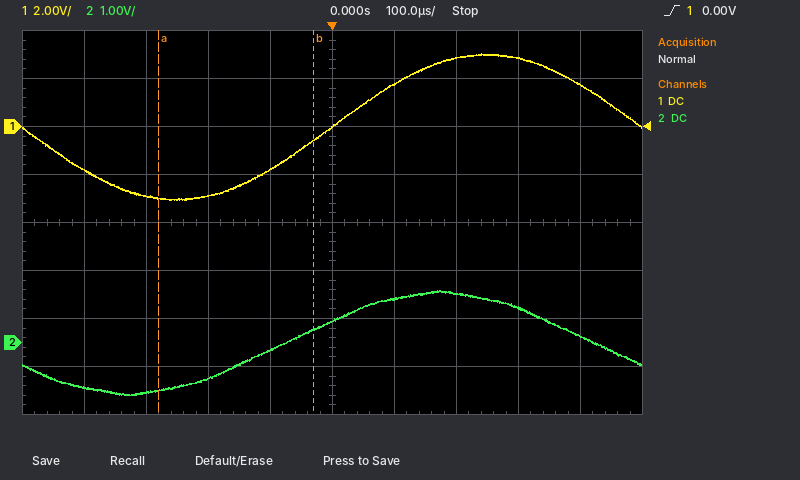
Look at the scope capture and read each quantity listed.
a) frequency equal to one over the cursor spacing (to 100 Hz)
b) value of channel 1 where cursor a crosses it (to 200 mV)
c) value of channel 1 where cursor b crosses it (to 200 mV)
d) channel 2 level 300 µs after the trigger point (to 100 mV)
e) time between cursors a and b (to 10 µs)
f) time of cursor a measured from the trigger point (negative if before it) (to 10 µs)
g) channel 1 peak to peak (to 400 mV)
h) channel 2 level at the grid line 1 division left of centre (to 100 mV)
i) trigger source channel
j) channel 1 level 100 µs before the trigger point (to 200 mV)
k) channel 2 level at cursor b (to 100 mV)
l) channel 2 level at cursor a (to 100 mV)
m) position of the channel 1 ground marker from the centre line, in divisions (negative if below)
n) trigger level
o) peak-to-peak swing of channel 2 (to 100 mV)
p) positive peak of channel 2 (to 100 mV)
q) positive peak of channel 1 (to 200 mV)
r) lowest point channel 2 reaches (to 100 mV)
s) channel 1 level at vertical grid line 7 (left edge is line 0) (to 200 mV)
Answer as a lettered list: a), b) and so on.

a) 4.0 kHz
b) -3.0 V
c) -600 mV
d) 700 mV
e) 250 µs
f) -280 µs
g) 6.0 V
h) -200 mV
i) channel 1
j) -1.8 V
k) 300 mV
l) -1.0 V
m) +2.0 div
n) 0.00 V
o) 2.2 V
p) 1.1 V
q) 3.0 V
r) -1.1 V
s) 2.8 V
